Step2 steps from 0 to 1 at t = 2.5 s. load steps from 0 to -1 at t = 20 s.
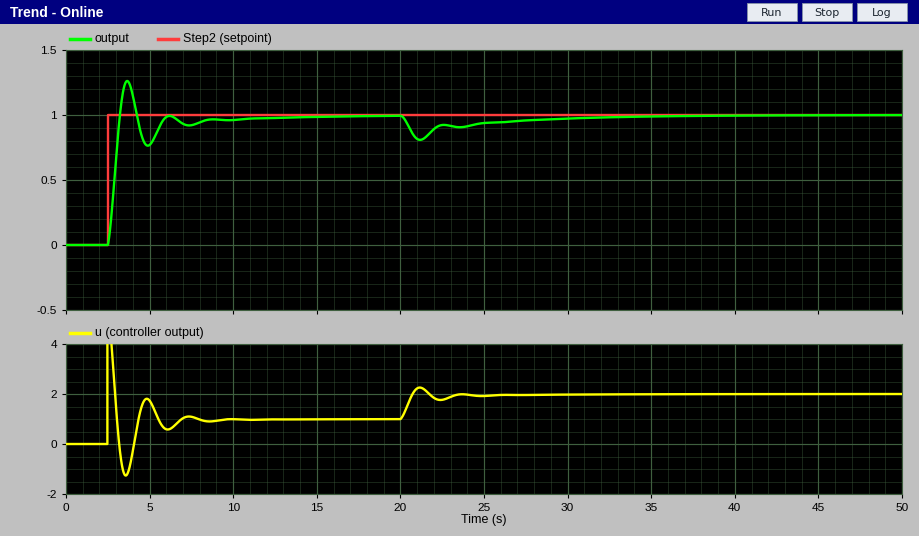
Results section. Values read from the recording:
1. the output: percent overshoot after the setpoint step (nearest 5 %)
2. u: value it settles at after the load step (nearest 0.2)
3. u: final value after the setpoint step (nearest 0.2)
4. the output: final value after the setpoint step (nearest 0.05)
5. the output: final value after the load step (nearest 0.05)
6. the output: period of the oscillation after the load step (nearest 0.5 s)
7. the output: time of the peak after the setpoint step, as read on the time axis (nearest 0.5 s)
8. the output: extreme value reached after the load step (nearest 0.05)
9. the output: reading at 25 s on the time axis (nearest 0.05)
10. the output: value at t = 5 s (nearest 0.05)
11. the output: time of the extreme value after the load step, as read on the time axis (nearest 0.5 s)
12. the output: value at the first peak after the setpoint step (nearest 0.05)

25 %
2.0
1.0
1.00
1.00
2.5 s
3.5 s
0.80
0.95
0.75
21.0 s
1.25
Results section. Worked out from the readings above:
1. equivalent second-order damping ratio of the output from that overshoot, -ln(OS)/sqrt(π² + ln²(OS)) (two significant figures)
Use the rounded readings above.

0.40
